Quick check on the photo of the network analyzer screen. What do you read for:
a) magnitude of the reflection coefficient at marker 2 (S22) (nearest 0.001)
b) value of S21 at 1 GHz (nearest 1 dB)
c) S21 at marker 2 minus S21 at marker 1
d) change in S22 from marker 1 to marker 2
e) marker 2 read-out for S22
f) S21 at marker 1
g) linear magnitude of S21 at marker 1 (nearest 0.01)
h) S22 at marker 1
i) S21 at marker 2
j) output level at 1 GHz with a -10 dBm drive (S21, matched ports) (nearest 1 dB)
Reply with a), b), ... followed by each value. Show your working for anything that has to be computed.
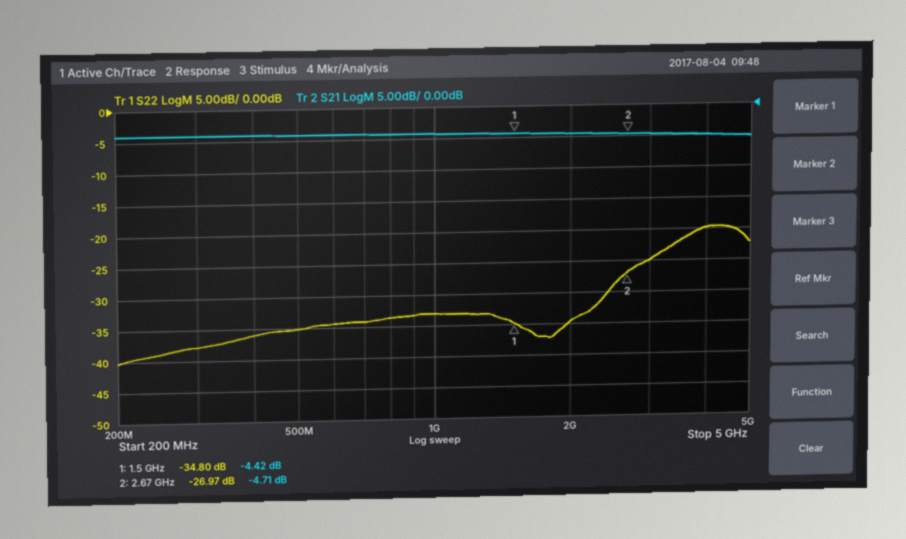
a) 10^(-26.97/20) ≈ 0.045
b) -4 dB
c) -4.71 − (-4.42) = -0.29 dB
d) -26.97 − (-34.8) = 7.83 dB
e) -26.97 dB
f) -4.42 dB
g) 10^(-4.42/20) ≈ 0.60
h) -34.80 dB
i) -4.71 dB
j) -10 dBm + (-4 dB) = -14 dBm
